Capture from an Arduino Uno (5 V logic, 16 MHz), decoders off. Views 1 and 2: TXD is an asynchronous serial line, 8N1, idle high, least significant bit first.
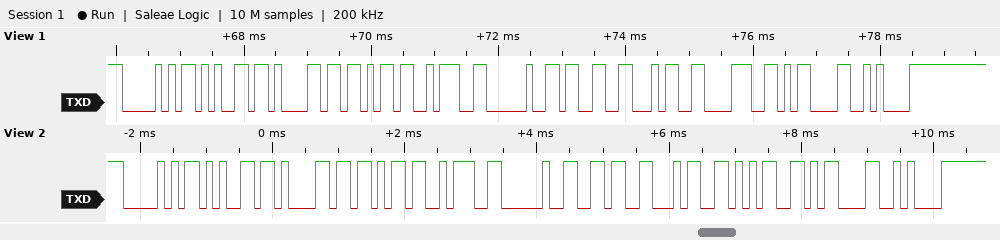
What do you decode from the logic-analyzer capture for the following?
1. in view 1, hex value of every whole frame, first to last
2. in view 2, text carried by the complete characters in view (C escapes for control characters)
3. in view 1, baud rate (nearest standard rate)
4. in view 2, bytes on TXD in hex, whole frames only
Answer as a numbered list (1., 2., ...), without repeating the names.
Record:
1. 50 65 61 6B 3A 20 33 34 38 0D 0A
2. "Peak: 645\r\n"
3. 9600 baud
4. 50 65 61 6B 3A 20 36 34 35 0D 0A
